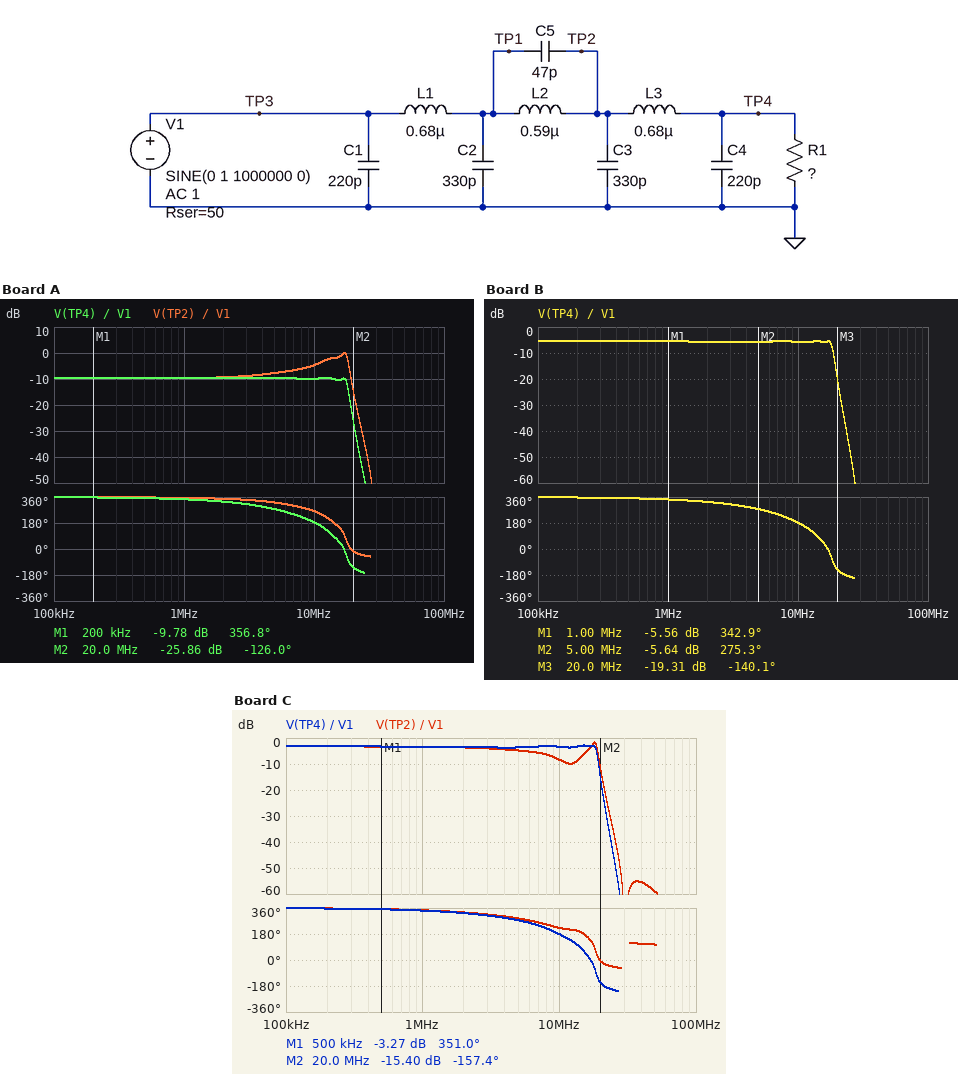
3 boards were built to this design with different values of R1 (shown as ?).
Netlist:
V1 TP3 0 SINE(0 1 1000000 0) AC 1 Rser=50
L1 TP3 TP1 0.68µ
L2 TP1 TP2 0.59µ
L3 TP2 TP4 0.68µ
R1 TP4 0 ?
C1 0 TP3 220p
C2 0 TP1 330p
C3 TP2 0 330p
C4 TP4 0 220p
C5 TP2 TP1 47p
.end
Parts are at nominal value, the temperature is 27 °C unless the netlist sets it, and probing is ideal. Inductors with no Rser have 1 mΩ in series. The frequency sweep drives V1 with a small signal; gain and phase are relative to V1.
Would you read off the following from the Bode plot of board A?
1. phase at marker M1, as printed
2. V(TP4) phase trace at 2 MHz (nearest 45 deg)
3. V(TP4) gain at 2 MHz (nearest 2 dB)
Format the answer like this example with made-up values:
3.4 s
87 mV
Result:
356.8 deg
315 deg
-10 dB
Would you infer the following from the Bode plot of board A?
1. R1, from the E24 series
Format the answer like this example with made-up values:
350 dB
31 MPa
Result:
24 Ω
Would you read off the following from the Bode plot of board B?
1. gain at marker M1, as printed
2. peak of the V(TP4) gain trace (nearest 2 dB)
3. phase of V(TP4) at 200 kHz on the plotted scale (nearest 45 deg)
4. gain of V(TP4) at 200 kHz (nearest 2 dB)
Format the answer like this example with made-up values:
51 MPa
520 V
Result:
-5.56 dB
-6 dB
360 deg
-6 dB
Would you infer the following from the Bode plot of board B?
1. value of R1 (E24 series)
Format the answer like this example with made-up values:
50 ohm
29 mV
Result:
56 Ω
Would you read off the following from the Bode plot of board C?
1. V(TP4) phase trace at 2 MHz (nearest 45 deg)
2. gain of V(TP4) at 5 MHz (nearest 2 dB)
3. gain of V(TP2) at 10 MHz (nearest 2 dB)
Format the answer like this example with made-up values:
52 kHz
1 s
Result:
315 deg
-4 dB
-8 dB
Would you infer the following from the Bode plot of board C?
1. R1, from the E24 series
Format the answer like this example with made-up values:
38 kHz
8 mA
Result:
110 Ω
